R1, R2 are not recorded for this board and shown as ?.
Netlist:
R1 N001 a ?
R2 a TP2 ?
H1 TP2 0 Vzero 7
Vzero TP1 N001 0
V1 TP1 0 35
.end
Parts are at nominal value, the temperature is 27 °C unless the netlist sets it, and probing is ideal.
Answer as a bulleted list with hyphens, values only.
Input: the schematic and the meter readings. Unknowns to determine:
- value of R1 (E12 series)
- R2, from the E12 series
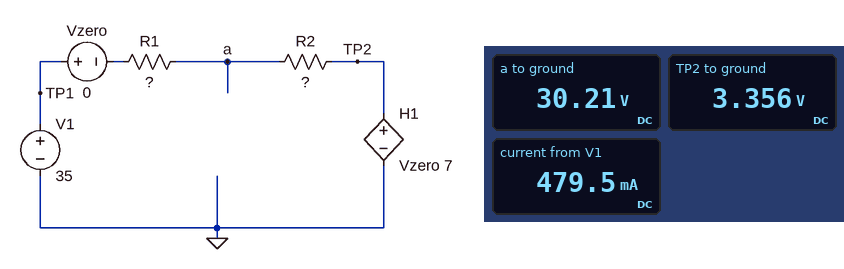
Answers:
- 10 Ω
- 56 Ω
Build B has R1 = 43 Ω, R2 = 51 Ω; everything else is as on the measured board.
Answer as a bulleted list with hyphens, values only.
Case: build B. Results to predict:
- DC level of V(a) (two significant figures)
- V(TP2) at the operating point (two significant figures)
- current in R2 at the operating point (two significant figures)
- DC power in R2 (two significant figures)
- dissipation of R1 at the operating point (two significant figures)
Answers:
- 20 V
- 2.4 V
- 350 mA
- 6.1 W
- 5.2 W
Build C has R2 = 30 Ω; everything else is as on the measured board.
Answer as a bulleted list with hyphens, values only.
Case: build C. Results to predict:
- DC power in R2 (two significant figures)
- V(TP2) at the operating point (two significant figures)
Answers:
- 17 W
- 5.2 V
